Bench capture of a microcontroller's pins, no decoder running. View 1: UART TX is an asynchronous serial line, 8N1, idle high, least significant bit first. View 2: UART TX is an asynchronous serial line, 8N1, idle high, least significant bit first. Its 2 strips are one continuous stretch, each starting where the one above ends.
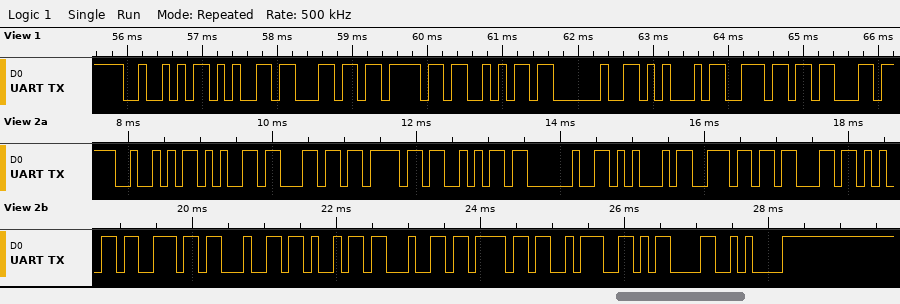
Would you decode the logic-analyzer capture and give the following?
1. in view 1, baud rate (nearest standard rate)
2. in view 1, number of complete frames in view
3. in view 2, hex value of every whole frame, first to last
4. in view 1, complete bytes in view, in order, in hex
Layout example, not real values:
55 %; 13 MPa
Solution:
9600 baud; 9; 52 65 6C 6F 6A 20 45 6E 63 65 6E 64 69 64 6F 3A 0D 0A; 52 65 6C 6F 6A 20 45 6E 63
